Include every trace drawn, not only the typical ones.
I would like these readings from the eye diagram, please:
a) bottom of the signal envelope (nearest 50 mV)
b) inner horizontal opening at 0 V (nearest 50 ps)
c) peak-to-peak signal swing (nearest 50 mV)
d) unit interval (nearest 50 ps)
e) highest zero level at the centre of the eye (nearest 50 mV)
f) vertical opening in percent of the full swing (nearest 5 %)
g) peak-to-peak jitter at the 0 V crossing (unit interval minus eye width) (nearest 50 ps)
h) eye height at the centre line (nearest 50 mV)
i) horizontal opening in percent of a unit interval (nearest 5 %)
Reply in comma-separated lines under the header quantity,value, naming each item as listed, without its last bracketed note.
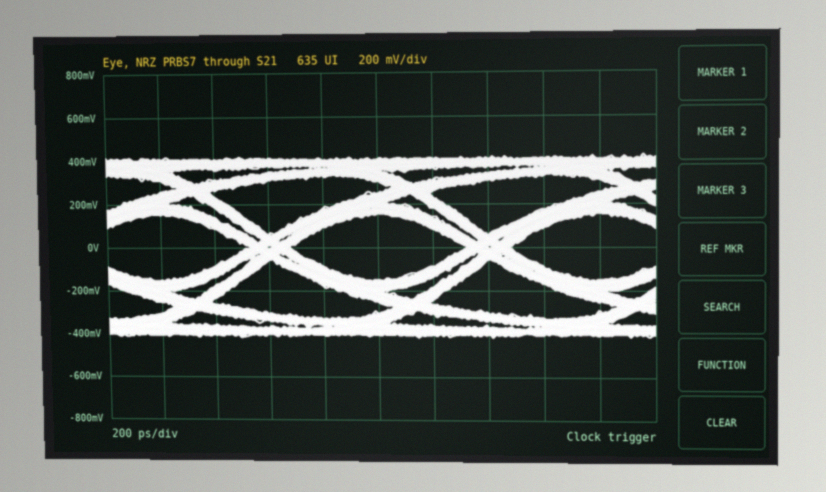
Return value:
quantity,value
bottom of the signal envelope,-400 mV
inner horizontal opening at 0 V,650 ps
peak-to-peak signal swing,850 mV
unit interval,800 ps
highest zero level at the centre of the eye,-150 mV
vertical opening in percent of the full swing,35 %
peak-to-peak jitter at the 0 V crossing (unit interval minus eye width),150 ps
eye height at the centre line,300 mV
horizontal opening in percent of a unit interval,80 %
